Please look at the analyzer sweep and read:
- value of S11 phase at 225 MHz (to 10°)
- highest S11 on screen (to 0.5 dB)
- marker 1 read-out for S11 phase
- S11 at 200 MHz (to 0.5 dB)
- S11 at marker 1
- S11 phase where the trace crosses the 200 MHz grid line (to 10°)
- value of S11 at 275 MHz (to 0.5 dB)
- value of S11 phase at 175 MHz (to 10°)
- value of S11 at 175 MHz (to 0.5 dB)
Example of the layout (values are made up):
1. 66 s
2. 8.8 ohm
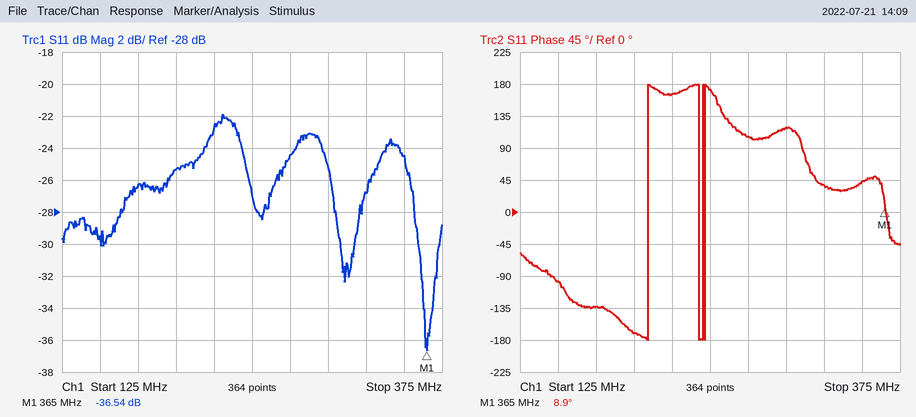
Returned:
1. 170°
2. -22.0 dB
3. 8.9°
4. -25.5 dB
5. -36.54 dB
6. -170°
7. -24.5 dB
8. -130°
9. -26.5 dB
